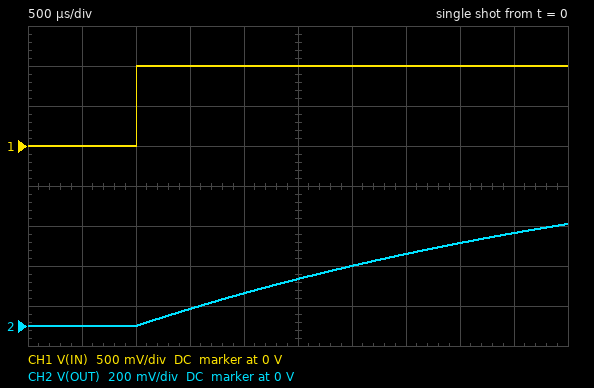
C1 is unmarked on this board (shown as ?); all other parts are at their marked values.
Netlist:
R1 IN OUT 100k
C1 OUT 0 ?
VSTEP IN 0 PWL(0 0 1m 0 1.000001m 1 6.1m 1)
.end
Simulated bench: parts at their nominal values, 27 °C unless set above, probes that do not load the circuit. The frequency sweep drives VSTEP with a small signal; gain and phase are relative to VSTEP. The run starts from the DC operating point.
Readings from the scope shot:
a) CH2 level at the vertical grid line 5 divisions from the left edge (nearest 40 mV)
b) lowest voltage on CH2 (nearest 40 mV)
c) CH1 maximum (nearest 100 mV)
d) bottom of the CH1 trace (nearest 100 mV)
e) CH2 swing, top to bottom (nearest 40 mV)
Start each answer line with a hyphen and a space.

- 240 mV
- 0 V
- 1.0 V
- 0 V
- 520 mV
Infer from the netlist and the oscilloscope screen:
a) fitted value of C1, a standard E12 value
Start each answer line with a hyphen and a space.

- 56 nF
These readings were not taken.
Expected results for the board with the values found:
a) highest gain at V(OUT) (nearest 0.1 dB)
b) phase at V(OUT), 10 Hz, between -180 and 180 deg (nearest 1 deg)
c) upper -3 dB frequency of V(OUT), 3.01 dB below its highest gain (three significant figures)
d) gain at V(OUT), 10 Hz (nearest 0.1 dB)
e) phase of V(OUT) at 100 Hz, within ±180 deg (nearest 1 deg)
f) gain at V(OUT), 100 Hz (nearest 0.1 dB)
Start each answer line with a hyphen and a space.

- 0 dB
- -19 deg
- 28.4 Hz
- -0.5 dB
- -74 deg
- -11.3 dB
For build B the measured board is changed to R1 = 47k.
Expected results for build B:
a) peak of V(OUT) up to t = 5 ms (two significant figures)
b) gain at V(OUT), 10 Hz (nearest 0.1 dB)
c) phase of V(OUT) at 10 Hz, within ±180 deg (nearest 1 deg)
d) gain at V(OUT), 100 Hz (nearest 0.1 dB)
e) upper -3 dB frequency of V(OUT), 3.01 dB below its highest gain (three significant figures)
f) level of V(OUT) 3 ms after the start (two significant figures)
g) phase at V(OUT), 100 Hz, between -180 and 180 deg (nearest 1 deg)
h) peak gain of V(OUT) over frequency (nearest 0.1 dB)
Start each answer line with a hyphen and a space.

- 780 mV
- -0.1 dB
- -9 deg
- -5.7 dB
- 60.5 Hz
- 530 mV
- -59 deg
- 0 dB
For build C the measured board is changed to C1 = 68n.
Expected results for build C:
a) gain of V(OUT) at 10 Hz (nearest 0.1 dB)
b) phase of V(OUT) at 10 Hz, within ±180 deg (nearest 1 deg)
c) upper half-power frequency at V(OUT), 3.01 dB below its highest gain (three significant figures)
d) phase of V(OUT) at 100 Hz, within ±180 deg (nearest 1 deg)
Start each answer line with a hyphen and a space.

- -0.7 dB
- -23 deg
- 23.4 Hz
- -77 deg
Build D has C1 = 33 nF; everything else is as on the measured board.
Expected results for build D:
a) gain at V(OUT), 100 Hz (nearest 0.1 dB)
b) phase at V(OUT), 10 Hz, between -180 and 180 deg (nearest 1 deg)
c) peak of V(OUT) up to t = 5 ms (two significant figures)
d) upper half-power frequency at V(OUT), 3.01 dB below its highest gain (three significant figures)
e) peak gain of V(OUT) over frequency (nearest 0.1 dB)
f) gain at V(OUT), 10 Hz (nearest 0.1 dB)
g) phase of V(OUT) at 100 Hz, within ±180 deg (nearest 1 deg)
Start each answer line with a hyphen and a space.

- -7.2 dB
- -12 deg
- 700 mV
- 48.2 Hz
- 0 dB
- -0.2 dB
- -64 deg
